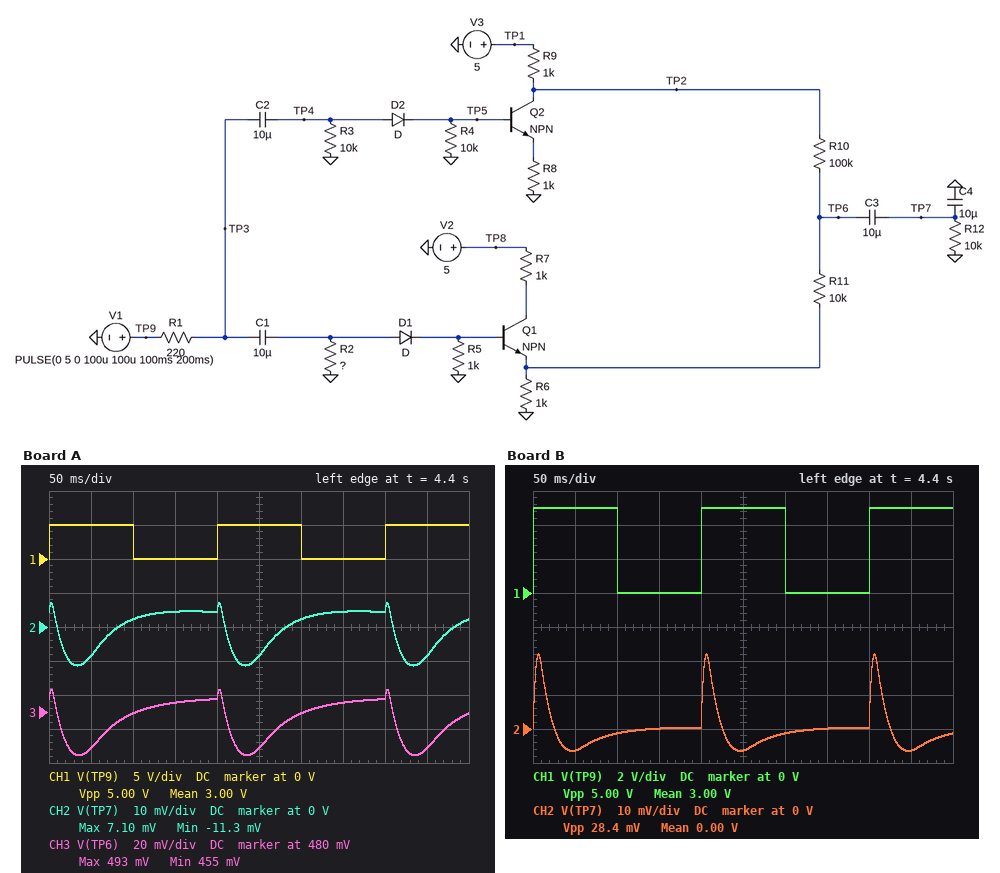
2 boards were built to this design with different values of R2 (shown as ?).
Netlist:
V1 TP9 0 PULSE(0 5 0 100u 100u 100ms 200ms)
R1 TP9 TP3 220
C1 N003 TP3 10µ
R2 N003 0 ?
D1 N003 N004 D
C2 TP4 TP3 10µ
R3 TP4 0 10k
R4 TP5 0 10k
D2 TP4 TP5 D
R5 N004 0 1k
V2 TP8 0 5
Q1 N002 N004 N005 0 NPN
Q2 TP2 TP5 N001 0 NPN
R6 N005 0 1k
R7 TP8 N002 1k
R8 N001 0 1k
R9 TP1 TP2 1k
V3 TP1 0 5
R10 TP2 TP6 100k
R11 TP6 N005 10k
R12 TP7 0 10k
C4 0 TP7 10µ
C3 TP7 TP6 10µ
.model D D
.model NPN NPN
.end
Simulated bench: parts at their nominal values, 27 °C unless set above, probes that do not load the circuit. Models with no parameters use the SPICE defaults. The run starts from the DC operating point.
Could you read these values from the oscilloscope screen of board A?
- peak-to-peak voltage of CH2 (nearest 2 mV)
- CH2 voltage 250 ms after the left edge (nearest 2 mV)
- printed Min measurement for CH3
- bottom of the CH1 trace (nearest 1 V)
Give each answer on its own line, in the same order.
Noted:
18 mV
-8 mV
455 mV
0 V
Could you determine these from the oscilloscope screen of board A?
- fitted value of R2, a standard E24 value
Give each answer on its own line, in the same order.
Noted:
20 kΩ
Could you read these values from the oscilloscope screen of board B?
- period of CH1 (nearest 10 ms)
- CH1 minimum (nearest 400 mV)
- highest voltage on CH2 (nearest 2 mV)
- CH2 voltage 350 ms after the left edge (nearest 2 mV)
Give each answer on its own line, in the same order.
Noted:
200 ms
0 V
22 mV
0 V
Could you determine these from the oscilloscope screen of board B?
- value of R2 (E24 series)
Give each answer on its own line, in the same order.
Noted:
12 kΩ
